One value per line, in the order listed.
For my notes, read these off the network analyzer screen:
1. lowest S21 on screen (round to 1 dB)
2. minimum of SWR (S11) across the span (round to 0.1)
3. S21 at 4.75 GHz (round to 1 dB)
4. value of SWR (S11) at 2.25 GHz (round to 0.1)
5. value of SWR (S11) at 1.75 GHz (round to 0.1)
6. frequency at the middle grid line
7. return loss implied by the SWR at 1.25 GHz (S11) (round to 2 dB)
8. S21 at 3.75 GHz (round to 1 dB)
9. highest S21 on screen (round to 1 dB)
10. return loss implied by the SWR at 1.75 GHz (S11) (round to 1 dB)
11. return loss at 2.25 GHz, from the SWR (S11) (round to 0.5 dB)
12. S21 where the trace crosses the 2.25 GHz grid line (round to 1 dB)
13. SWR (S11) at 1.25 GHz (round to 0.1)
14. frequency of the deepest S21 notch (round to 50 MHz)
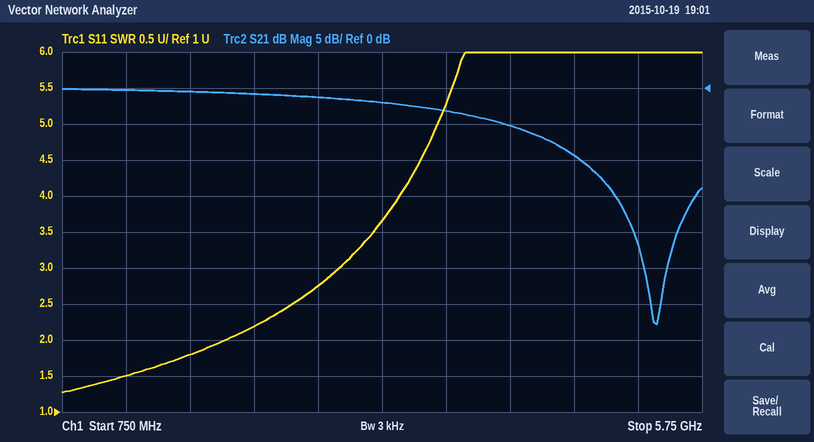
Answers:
-33 dB
1.3
-9 dB
2.2
1.8
3.25 GHz
14 dB
-3 dB
0 dB
11 dB
8.5 dB
-1 dB
1.5
5.40 GHz
